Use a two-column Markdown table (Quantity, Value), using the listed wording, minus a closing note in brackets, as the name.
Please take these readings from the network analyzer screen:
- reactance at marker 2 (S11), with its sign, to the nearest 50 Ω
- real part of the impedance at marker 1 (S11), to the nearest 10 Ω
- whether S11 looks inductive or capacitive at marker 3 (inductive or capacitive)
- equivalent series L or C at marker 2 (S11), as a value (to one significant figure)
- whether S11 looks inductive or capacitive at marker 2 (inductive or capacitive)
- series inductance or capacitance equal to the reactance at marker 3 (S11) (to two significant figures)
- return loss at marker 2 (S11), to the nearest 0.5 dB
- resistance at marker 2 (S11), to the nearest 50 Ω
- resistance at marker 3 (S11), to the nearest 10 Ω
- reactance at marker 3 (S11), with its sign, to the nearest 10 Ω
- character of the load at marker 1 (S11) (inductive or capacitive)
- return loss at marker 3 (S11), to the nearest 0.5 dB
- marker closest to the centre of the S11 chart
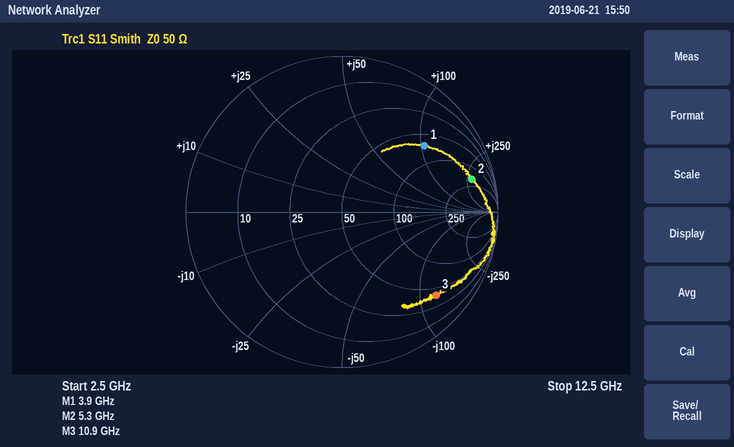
| Quantity | Value |
|---|---|
| reactance at marker 2 (S11), with its sign, to the nearest 50 Ω | +300 Ω |
| real part of the impedance at marker 1 (S11), to the nearest 10 Ω | 70 Ω |
| whether S11 looks inductive or capacitive at marker 3 | capacitive |
| equivalent series L or C at marker 2 (S11), as a value | 9 nH |
| whether S11 looks inductive or capacitive at marker 2 | inductive |
| series inductance or capacitance equal to the reactance at marker 3 (S11) | 120 fF |
| return loss at marker 2 (S11), to the nearest 0.5 dB | 1.5 dB |
| resistance at marker 2 (S11), to the nearest 50 Ω | 200 Ω |
| resistance at marker 3 (S11), to the nearest 10 Ω | 40 Ω |
| reactance at marker 3 (S11), with its sign, to the nearest 10 Ω | -120 Ω |
| character of the load at marker 1 (S11) | inductive |
| return loss at marker 3 (S11), to the nearest 0.5 dB | 2.0 dB |
| marker closest to the centre of the S11 chart | marker 1 |
